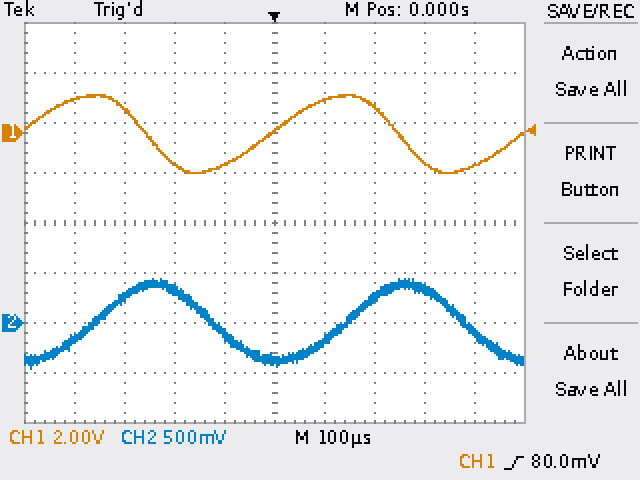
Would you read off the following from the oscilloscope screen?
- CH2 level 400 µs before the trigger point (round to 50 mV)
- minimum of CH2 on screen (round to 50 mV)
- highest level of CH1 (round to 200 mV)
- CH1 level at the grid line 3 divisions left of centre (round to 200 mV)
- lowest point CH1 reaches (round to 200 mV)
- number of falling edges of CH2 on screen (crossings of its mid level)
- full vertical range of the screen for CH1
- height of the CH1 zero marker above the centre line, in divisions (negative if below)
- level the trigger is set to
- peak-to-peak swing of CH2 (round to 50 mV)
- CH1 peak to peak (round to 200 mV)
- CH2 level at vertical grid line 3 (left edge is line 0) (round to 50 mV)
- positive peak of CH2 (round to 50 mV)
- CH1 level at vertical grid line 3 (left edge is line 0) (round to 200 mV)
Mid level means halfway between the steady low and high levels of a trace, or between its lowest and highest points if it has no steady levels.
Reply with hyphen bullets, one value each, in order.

- -150 mV
- -450 mV
- 1.6 V
- 1.0 V
- -1.6 V
- 2
- 16 V
- +1.8 div
- 80.0 mV
- 900 mV
- 3.2 V
- 350 mV
- 450 mV
- -1.2 V
